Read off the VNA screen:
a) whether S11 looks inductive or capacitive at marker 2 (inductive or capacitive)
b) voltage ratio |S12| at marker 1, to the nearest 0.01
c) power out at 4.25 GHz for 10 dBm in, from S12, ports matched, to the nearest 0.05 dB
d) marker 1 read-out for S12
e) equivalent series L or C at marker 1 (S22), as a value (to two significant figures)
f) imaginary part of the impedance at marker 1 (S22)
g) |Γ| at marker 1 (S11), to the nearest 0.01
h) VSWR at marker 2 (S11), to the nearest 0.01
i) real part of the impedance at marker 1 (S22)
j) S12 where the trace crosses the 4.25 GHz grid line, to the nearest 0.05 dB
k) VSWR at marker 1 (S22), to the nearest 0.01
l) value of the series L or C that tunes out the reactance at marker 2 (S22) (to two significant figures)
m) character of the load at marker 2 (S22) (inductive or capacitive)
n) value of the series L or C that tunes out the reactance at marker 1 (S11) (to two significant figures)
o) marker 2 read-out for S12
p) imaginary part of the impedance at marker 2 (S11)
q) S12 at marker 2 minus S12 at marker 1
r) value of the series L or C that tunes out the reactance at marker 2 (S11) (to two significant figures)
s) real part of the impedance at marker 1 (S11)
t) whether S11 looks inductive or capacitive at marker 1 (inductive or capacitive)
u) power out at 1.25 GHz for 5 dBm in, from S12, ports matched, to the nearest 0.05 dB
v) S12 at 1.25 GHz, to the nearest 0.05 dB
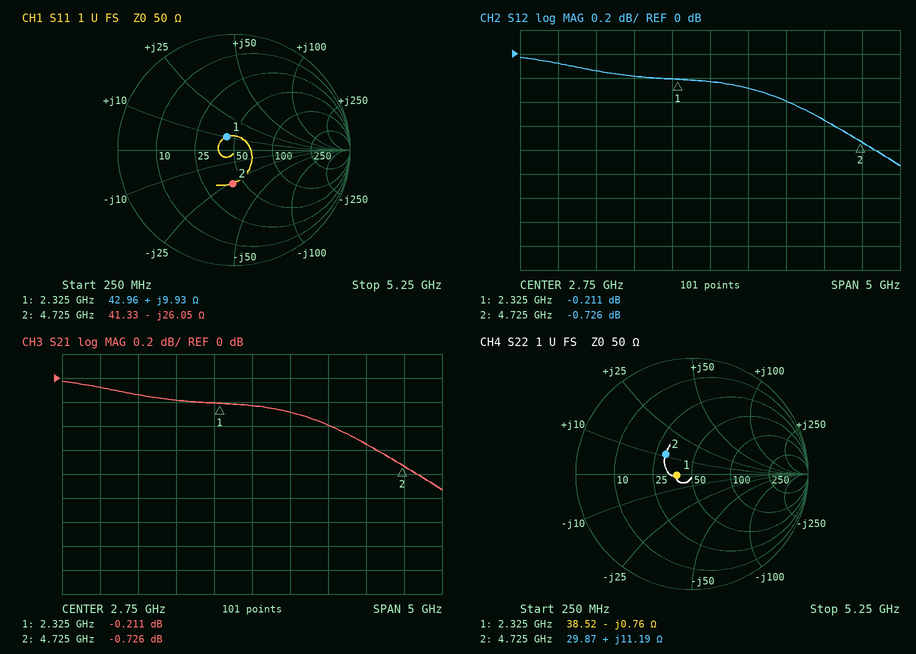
capacitive
0.98
9.45 dBm
-0.211 dB
90 pF
-0.76 Ω
0.13
1.81
38.52 Ω
-0.55 dB
1.30
3.0 pF
inductive
6.9 pF
-0.726 dB
-26.05 Ω
-0.515 dB
880 pH
42.96 Ω
inductive
4.85 dBm
-0.15 dB
